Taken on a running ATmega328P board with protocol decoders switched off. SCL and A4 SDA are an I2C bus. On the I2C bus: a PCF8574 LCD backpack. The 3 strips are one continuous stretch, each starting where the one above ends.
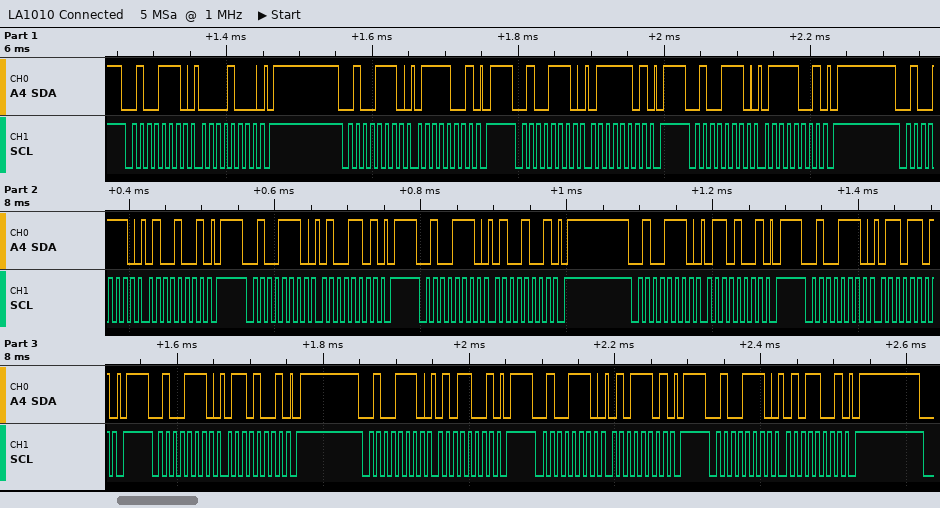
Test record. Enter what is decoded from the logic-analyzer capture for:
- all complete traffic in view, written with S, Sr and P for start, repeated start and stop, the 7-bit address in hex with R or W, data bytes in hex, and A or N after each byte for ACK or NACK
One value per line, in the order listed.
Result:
S 27W A 08 A P S 27W A 79 A P S 27W A 7D A P S 27W A 79 A P S 27W A 49 A P S 27W A 4D A P S 27W A 49 A P S 27W A 69 A P S 27W A 6D A P S 27W A 69 A P S 27W A 59 A P S 27W A 5D A P S 27W A 59 A P
